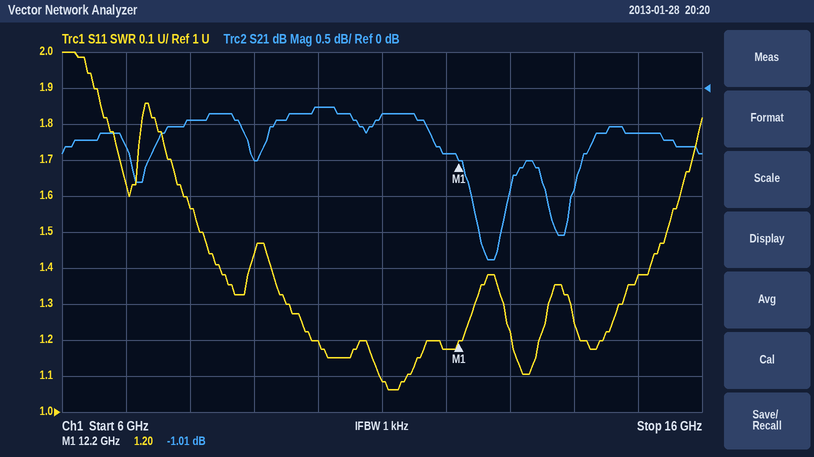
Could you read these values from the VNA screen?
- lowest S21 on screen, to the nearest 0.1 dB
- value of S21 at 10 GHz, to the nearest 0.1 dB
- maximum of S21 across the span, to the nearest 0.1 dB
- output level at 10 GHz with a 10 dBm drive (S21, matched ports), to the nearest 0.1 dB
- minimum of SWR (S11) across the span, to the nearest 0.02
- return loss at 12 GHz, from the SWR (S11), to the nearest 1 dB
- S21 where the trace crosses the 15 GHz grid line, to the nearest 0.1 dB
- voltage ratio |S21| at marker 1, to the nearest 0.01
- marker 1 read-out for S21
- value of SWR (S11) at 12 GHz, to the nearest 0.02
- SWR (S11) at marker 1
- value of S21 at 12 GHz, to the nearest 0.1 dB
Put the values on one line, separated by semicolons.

-2.4 dB; -0.3 dB; -0.3 dB; 9.7 dBm; 1.06; 22 dB; -0.6 dB; 0.89; -1.01 dB; 1.18; 1.20; -0.9 dB
